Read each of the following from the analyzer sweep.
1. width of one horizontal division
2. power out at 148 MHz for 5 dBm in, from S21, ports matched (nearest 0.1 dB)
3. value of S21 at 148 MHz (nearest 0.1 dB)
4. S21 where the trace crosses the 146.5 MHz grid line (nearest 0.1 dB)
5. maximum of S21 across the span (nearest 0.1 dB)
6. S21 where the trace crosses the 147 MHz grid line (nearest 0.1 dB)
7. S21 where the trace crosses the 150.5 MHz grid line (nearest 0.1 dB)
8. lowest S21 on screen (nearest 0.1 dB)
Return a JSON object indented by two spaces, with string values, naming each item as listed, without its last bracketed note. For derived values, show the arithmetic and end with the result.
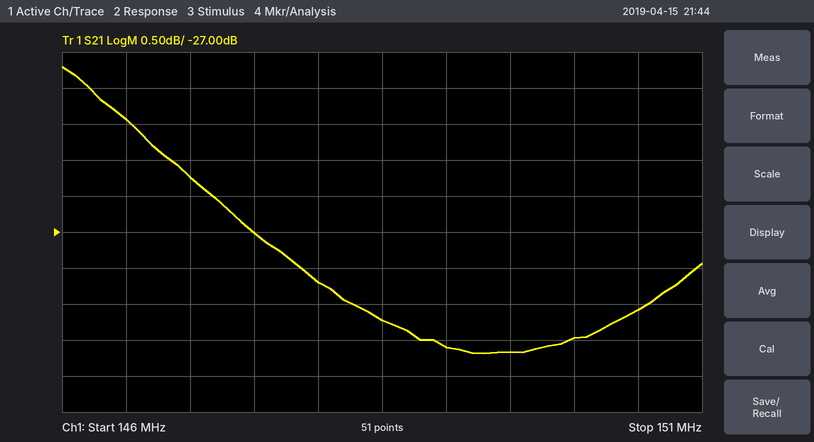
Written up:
{
  "width of one horizontal division": "500 kHz",
  "power out at 148 MHz for 5 dBm in, from S21, ports matched": "5 dBm + (-27.7 dB) = -22.7 dBm",
  "value of S21 at 148 MHz": "-27.7 dB",
  "S21 where the trace crosses the 146.5 MHz grid line": "-25.4 dB",
  "maximum of S21 across the span": "-24.7 dB",
  "S21 where the trace crosses the 147 MHz grid line": "-26.2 dB",
  "S21 where the trace crosses the 150.5 MHz grid line": "-28.1 dB",
  "lowest S21 on screen": "-28.7 dB"
}
